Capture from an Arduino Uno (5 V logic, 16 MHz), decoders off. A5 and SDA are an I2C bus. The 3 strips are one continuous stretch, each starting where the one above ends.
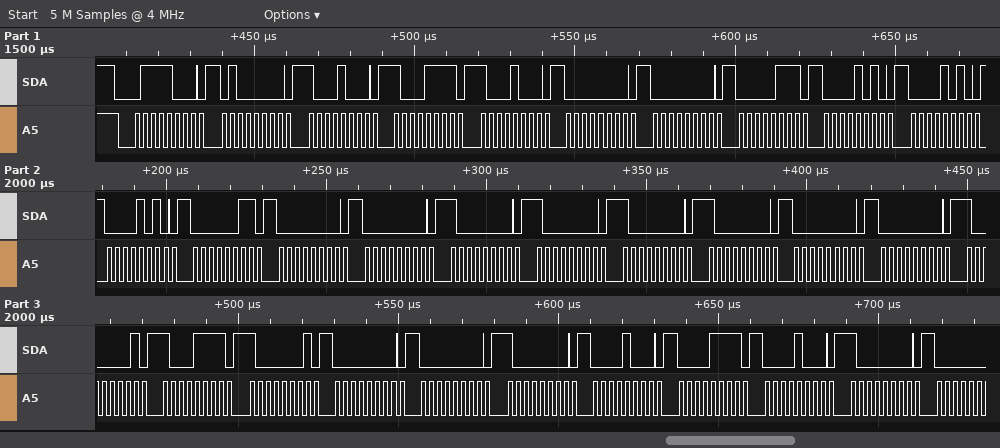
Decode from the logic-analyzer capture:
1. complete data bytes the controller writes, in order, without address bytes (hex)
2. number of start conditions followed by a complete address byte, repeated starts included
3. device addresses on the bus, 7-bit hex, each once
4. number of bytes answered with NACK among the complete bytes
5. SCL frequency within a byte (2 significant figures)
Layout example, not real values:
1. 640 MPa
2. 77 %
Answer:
1. 40 88 8F 88 00 00 07 0A 0A 0A 03 00 00 80 80 80 80 00 00 81 8F 81 00 00 80 08 0F 08 80
2. 1
3. 0x3C
4. 0
5. 400 kHz
